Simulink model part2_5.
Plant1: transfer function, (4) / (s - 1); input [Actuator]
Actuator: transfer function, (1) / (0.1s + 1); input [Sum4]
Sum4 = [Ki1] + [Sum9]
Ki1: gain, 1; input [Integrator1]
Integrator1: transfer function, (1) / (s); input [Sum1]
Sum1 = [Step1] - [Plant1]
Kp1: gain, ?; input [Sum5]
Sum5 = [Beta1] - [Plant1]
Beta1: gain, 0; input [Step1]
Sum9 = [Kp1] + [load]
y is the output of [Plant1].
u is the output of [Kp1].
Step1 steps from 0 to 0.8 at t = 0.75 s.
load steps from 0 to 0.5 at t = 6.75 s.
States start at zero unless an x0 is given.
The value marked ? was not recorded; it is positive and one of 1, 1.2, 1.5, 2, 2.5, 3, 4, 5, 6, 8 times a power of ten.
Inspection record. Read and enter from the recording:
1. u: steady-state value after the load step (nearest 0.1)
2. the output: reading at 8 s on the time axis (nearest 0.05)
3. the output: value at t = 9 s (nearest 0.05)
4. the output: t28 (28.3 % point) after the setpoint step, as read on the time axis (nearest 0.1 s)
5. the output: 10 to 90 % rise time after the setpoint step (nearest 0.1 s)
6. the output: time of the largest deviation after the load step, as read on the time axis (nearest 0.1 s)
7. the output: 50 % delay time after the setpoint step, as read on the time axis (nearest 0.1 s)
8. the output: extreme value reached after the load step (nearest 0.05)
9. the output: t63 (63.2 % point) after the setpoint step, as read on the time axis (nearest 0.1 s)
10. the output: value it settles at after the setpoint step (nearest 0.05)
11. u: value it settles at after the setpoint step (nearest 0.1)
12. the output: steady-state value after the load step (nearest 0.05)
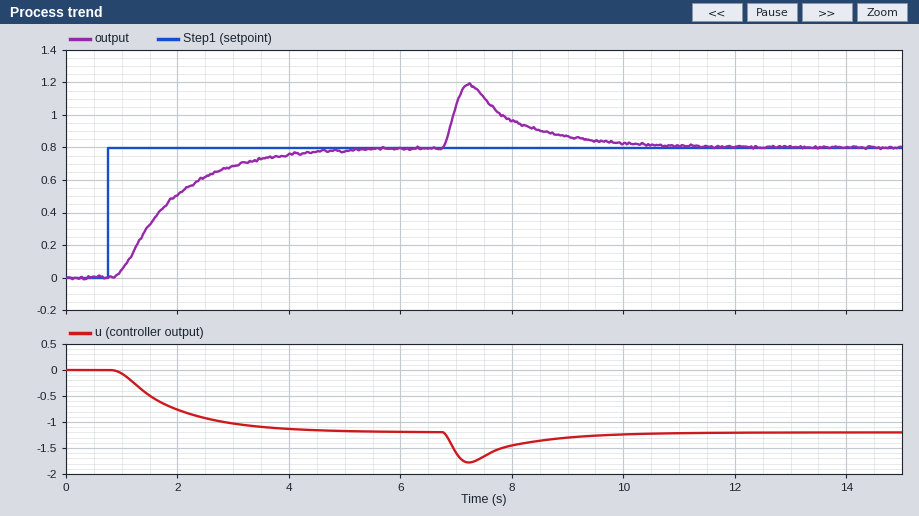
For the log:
-1.2
0.95
0.85
1.3 s
2.3 s
7.2 s
1.7 s
1.20
2.0 s
0.80
-1.2
0.80
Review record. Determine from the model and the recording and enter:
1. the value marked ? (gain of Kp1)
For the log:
1.5
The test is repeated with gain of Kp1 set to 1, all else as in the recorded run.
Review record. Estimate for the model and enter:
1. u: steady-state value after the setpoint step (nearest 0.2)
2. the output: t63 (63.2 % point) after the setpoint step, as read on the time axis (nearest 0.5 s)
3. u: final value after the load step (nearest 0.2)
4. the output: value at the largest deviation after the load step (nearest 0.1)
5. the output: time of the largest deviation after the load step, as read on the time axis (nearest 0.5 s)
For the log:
-0.8
1.5 s
-0.8
1.3
7.5 s
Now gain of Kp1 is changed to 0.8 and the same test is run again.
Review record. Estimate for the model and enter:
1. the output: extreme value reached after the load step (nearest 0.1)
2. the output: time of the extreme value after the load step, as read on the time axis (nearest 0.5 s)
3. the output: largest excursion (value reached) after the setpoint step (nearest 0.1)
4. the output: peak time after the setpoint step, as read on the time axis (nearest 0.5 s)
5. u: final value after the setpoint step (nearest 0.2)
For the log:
1.4
7.5 s
0.9
2.5 s
-0.6
